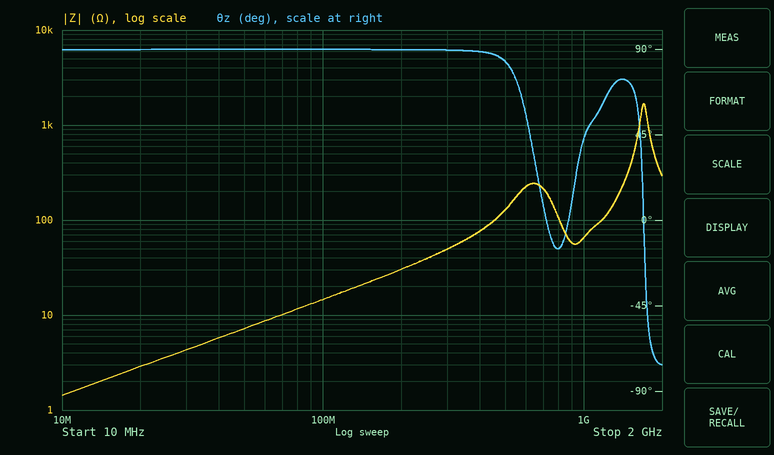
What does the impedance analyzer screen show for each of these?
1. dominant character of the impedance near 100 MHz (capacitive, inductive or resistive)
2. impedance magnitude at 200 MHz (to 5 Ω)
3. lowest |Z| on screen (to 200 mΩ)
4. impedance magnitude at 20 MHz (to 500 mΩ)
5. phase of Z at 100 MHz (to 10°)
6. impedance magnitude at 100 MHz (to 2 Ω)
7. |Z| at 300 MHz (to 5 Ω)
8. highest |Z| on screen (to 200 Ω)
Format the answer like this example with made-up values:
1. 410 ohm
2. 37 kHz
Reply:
1. inductive
2. 30 Ω
3. 1.4 Ω
4. 3.0 Ω
5. 90°
6. 14 Ω
7. 50 Ω
8. 1.6 kΩ
